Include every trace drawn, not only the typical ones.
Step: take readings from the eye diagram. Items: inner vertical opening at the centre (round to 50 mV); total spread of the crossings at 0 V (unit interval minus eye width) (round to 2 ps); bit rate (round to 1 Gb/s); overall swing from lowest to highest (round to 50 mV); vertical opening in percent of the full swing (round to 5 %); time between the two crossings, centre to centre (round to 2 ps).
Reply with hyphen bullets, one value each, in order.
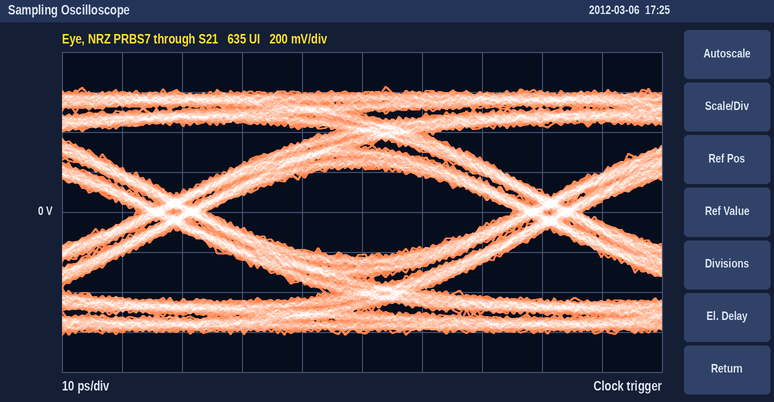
- 450 mV
- 12 ps
- 16 Gb/s
- 1.25 V
- 35 %
- 62 ps
